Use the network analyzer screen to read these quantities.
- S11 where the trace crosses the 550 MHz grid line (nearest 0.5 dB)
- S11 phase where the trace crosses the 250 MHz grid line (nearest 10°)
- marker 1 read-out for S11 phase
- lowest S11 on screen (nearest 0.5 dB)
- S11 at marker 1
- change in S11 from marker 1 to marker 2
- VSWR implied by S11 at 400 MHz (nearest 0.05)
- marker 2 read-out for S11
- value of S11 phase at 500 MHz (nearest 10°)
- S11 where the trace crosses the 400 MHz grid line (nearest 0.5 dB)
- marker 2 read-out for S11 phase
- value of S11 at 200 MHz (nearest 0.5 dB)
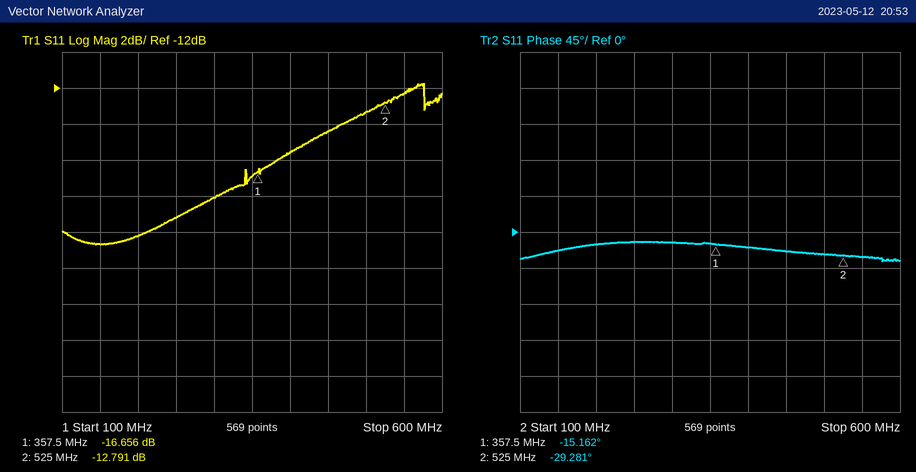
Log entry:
-12.5 dB
-10°
-15.162°
-20.5 dB
-16.656 dB
3.865 dB
1.40
-12.791 dB
-30°
-15.5 dB
-29.281°
-20.0 dB
